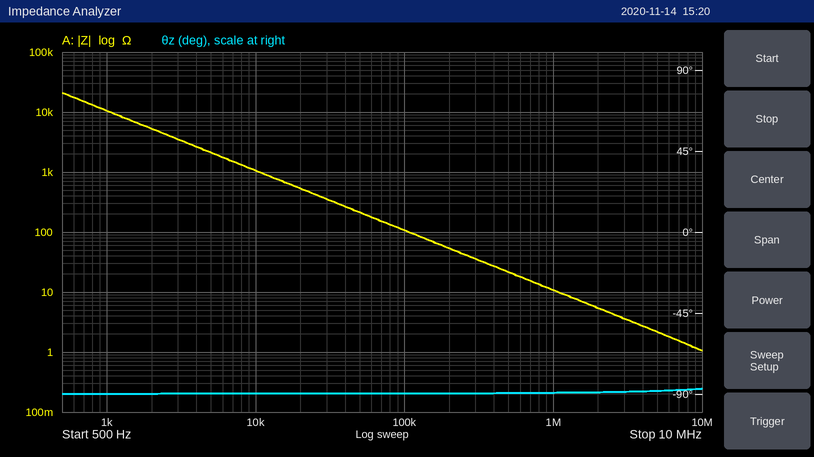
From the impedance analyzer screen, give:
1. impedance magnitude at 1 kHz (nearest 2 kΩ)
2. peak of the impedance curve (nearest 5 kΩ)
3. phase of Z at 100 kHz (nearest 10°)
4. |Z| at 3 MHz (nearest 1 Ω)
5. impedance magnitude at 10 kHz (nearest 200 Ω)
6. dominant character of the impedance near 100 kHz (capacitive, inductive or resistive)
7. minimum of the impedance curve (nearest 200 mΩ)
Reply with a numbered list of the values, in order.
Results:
1. 10 kΩ
2. 20 kΩ
3. -90°
4. 4 Ω
5. 1.0 kΩ
6. capacitive
7. 1.0 Ω
